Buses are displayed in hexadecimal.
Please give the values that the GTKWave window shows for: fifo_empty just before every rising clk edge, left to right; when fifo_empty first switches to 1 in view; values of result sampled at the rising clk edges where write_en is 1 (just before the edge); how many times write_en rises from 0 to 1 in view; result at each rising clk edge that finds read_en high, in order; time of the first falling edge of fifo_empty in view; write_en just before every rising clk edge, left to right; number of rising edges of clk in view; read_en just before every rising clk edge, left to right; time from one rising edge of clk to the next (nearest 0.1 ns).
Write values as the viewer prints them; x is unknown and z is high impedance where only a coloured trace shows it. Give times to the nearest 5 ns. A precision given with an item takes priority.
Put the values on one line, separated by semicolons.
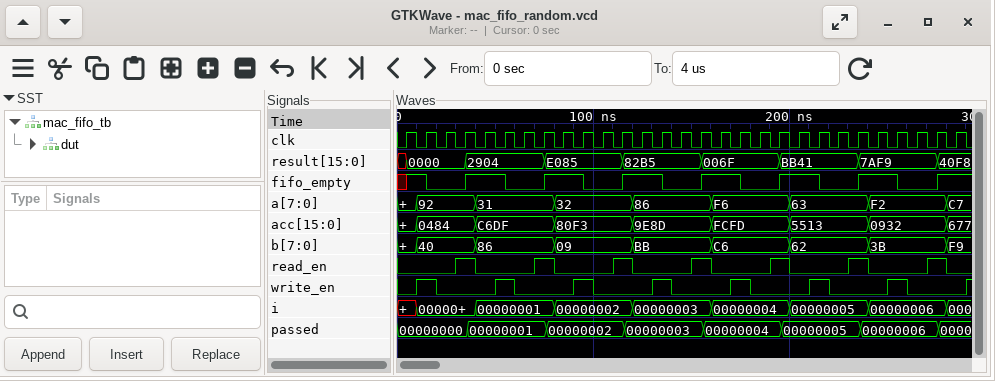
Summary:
x 1 0 0 1 1 0 0 1 1 0 0 1 1 0 0 1 1 0 0 1 1 0 0 1 1 0 0 1; 5 ns; 0000, 2904, E085, 82B5, 006F, BB41, 7AF9; 8; 0000, 2904, E085, 82B5, 006F, BB41, 7AF9; 15 ns; 0 1 0 0 0 1 0 0 0 1 0 0 0 1 0 0 0 1 0 0 0 1 0 0 0 1 0 0 0; 29; 0 0 0 1 0 0 0 1 0 0 0 1 0 0 0 1 0 0 0 1 0 0 0 1 0 0 0 1 0; 10 ns
